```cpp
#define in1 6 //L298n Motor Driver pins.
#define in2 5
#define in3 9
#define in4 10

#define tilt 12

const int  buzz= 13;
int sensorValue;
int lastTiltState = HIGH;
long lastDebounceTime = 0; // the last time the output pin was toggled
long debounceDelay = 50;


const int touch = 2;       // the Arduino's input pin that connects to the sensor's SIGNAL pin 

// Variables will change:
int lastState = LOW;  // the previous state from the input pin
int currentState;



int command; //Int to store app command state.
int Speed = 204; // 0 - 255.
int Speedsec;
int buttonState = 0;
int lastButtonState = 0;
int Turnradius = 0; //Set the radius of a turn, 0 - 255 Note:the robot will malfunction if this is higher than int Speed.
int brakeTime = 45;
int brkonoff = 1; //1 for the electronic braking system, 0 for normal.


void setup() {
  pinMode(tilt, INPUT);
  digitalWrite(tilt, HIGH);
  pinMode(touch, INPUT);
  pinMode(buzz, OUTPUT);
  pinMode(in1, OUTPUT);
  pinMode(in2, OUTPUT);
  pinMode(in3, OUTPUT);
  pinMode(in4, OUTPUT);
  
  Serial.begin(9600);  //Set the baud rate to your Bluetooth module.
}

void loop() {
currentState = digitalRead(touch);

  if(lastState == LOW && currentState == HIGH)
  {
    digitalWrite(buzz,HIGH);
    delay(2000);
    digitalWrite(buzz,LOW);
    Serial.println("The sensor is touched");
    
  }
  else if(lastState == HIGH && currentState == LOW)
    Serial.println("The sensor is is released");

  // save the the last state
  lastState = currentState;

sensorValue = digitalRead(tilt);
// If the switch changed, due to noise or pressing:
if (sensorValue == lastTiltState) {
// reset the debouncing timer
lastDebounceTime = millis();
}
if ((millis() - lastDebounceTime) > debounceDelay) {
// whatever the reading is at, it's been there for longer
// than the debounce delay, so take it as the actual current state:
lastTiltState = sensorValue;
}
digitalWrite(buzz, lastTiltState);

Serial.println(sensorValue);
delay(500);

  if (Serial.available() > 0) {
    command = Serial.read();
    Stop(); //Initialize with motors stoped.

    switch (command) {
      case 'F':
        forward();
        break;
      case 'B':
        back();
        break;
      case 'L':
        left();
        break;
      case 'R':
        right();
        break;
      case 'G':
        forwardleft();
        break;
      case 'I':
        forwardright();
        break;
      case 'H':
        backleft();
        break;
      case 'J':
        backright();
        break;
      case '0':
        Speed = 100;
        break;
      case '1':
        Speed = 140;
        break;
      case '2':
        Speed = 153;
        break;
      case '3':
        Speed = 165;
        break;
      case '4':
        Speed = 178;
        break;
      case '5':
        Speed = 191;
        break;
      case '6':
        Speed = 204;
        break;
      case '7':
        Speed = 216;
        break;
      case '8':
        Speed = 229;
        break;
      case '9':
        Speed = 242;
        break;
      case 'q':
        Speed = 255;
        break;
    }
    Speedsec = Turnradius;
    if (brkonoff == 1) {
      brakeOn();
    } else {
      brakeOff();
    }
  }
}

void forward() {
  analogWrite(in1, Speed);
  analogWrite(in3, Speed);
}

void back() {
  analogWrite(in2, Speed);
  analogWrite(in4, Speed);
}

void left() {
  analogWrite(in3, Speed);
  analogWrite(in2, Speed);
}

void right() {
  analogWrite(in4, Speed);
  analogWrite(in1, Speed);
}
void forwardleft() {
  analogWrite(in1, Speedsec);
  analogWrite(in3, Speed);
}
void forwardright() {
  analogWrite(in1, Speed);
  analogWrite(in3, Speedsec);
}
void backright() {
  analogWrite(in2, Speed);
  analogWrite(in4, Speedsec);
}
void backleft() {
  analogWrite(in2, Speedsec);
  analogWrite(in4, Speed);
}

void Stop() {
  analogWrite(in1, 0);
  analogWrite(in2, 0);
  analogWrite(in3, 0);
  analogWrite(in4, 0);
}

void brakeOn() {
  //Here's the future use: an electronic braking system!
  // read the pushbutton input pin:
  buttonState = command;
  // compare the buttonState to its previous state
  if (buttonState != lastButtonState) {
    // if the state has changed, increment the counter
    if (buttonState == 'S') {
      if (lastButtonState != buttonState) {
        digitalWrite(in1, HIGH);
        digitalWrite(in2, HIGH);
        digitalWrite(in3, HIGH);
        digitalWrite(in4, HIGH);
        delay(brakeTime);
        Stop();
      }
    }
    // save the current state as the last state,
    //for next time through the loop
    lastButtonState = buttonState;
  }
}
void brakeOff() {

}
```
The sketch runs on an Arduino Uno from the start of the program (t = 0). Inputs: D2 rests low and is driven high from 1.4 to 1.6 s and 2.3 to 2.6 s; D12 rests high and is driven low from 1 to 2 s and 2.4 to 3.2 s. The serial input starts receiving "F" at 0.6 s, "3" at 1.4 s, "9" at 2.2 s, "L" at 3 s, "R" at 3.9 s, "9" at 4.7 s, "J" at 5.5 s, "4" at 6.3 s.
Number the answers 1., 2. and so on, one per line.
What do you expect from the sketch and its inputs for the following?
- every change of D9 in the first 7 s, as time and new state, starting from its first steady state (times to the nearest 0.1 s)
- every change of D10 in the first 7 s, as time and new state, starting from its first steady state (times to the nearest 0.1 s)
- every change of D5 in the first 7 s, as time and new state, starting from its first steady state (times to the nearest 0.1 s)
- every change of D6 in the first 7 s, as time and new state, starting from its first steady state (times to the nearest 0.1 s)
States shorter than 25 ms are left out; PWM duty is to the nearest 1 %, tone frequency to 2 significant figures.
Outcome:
1. 0 s low; 1 s PWM 80 %; 1.5 s low; 4.5 s PWM 95 %; 5 s low
2. 0 s low; 5 s PWM 95 %; 5.5 s low
3. 0 s low; 4.5 s PWM 95 %; 5 s low; 6 s PWM 95 %; 6.5 s low
4. 0 s low; 1 s PWM 80 %; 1.5 s low; 5 s PWM 95 %; 5.5 s low
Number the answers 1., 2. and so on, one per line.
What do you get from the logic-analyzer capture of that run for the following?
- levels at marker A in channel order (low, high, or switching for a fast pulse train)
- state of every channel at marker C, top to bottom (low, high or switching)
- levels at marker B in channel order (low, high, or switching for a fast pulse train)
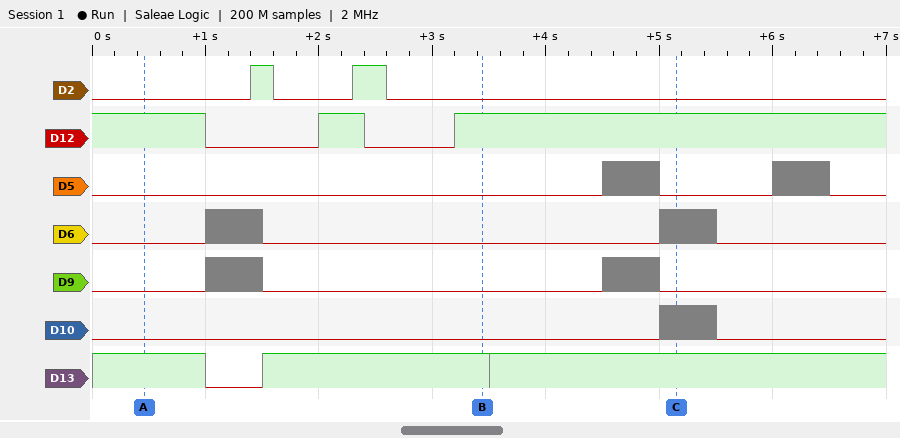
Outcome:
1. D2 low, D12 high, D5 low, D6 low, D9 low, D10 low, D13 high
2. D2 low, D12 high, D5 low, D6 switching, D9 low, D10 switching, D13 high
3. D2 low, D12 high, D5 low, D6 low, D9 low, D10 low, D13 high
